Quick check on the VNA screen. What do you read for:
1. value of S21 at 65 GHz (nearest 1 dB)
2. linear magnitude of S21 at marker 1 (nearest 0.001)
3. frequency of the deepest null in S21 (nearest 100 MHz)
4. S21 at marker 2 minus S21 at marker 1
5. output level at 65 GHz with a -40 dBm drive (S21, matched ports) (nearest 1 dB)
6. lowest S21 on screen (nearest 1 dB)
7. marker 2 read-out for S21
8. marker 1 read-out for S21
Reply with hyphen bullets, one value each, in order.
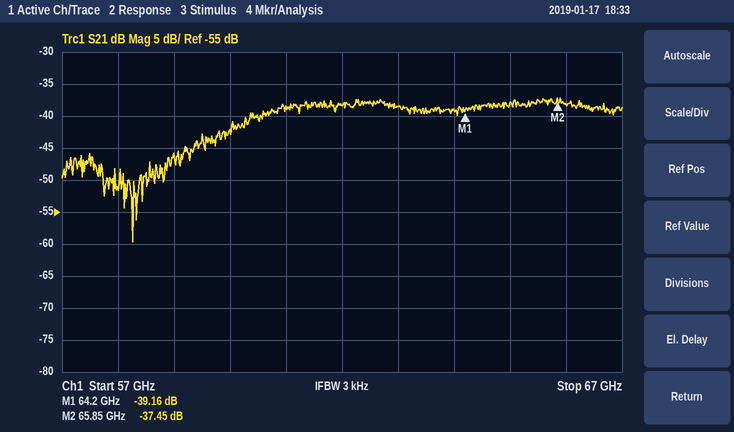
- -38 dB
- 0.011
- 58.3 GHz
- 1.71 dB
- -78 dBm
- -60 dB
- -37.45 dB
- -39.16 dB
